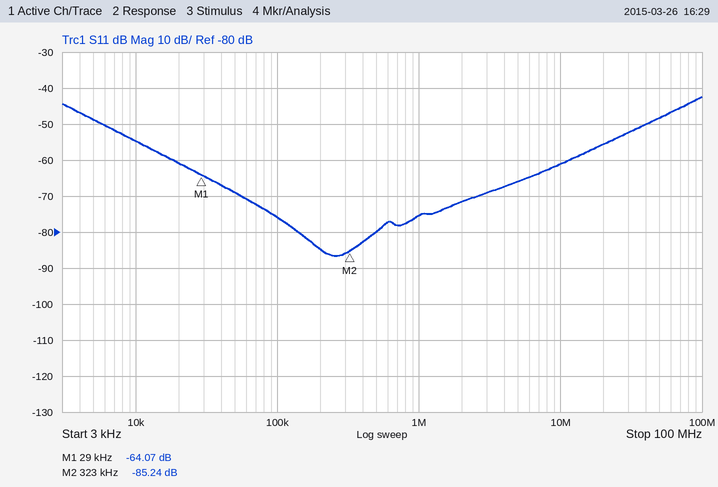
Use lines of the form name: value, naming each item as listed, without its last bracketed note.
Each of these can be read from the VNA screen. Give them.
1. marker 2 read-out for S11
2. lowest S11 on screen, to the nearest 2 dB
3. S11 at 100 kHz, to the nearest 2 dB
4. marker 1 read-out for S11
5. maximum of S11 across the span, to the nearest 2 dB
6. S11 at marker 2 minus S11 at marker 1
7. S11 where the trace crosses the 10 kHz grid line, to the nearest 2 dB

marker 2 read-out for S11: -85.24 dB
lowest S11 on screen, to the nearest 2 dB: -86 dB
S11 at 100 kHz, to the nearest 2 dB: -76 dB
marker 1 read-out for S11: -64.07 dB
maximum of S11 across the span, to the nearest 2 dB: -42 dB
S11 at marker 2 minus S11 at marker 1: -21.17 dB
S11 where the trace crosses the 10 kHz grid line, to the nearest 2 dB: -54 dB
